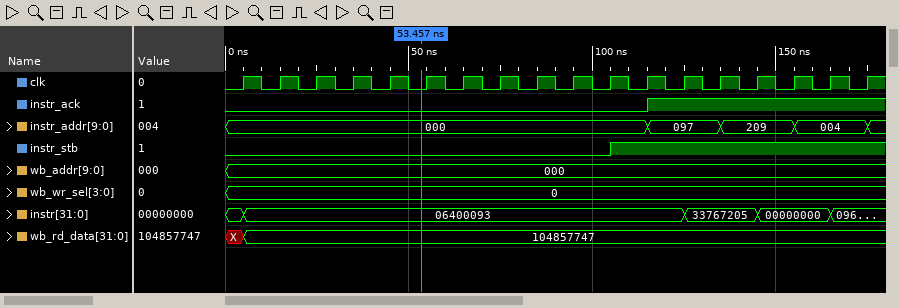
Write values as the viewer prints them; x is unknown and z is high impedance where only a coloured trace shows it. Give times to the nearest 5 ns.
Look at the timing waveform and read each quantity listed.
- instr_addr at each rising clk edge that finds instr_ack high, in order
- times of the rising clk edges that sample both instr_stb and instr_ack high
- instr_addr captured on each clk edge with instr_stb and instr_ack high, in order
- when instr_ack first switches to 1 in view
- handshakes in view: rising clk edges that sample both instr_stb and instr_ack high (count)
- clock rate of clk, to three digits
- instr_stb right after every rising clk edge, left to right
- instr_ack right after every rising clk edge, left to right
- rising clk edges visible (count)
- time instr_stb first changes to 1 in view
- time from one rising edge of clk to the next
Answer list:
097, 097, 209, 209, 004, 004
125 ns, 135 ns, 145 ns, 155 ns, 165 ns, 175 ns
097, 097, 209, 209, 004, 004
115 ns
6
100 MHz
0 0 0 0 0 0 0 0 0 0 1 1 1 1 1 1 1 1
0 0 0 0 0 0 0 0 0 0 0 1 1 1 1 1 1 1
18
105 ns
10 ns
